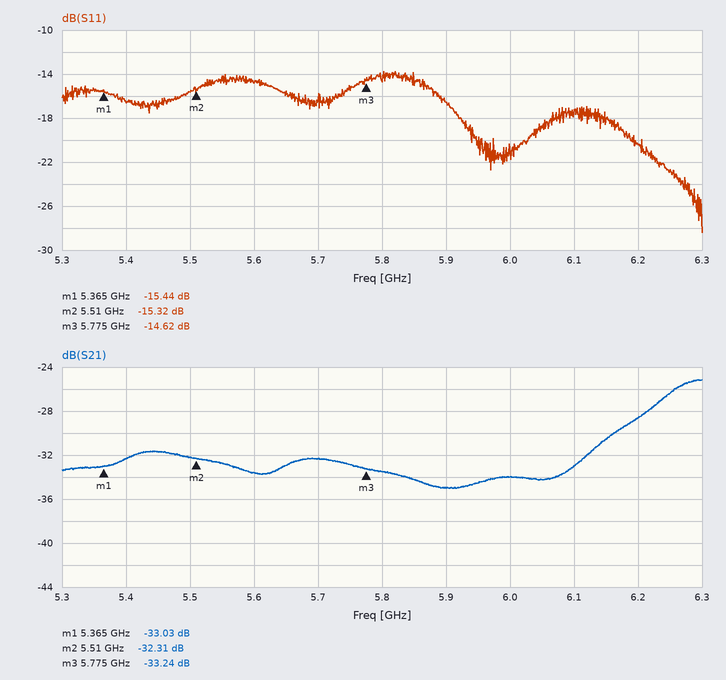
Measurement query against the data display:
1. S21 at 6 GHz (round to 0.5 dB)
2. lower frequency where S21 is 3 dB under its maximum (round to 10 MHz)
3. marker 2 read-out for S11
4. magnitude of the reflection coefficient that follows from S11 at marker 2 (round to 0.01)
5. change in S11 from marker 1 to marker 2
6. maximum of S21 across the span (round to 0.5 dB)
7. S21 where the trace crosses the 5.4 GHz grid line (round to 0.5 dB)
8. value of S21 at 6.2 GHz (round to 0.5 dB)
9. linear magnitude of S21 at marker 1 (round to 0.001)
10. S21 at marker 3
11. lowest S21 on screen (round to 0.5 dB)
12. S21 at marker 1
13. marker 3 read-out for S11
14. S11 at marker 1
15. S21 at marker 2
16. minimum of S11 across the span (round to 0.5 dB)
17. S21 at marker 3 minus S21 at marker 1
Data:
-34.0 dB
6.21 GHz
-15.32 dB
0.17
0.12 dB
-25.0 dB
-32.5 dB
-28.5 dB
0.022
-33.24 dB
-35.0 dB
-33.03 dB
-14.62 dB
-15.44 dB
-32.31 dB
-28.5 dB
-0.21 dB
